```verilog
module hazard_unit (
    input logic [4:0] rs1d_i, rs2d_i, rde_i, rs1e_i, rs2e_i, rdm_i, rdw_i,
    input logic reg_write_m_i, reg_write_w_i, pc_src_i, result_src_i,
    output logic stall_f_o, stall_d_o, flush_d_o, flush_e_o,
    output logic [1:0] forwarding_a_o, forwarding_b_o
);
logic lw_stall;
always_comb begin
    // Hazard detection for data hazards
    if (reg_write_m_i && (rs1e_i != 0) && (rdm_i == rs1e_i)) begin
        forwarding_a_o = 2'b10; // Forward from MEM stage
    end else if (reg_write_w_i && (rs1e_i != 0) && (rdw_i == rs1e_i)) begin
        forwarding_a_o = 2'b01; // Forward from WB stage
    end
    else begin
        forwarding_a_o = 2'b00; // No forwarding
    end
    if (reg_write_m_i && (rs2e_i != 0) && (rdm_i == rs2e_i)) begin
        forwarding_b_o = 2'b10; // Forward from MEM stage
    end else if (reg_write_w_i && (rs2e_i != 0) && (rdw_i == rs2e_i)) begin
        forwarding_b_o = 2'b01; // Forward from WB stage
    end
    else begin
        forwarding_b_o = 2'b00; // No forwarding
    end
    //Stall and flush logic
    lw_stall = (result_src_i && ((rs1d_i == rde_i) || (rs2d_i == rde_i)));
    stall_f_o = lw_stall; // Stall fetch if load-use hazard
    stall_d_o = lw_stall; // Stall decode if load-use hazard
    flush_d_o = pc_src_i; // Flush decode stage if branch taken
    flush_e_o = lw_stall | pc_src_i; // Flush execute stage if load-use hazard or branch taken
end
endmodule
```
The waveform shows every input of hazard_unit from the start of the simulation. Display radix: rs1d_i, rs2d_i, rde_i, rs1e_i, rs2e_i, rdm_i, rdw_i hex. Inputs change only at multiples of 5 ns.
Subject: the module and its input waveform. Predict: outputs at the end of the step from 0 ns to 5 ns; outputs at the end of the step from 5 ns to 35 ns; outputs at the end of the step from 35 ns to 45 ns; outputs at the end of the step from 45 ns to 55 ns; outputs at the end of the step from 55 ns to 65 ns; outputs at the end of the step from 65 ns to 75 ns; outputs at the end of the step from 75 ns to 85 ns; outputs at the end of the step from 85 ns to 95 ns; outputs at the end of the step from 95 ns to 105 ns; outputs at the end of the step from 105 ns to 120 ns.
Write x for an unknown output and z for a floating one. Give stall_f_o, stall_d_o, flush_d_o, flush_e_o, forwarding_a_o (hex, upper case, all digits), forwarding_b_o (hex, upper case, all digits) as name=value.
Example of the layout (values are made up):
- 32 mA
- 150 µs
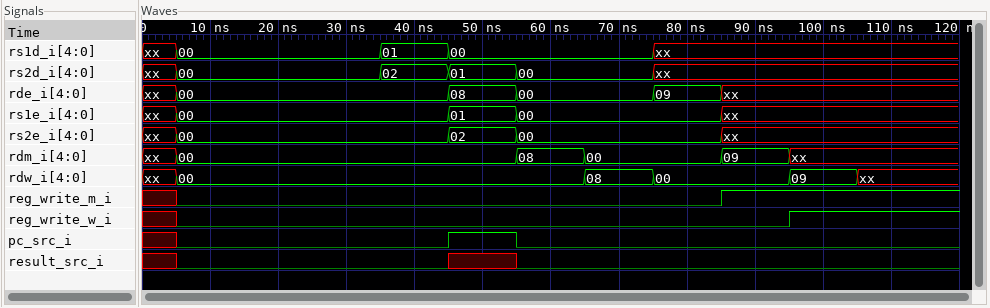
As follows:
- stall_f_o=x, stall_d_o=x, flush_d_o=x, flush_e_o=x, forwarding_a_o=0, forwarding_b_o=0
- stall_f_o=0, stall_d_o=0, flush_d_o=0, flush_e_o=0, forwarding_a_o=0, forwarding_b_o=0
- stall_f_o=0, stall_d_o=0, flush_d_o=0, flush_e_o=0, forwarding_a_o=0, forwarding_b_o=0
- stall_f_o=0, stall_d_o=0, flush_d_o=1, flush_e_o=1, forwarding_a_o=0, forwarding_b_o=0
- stall_f_o=0, stall_d_o=0, flush_d_o=0, flush_e_o=0, forwarding_a_o=0, forwarding_b_o=0
- stall_f_o=0, stall_d_o=0, flush_d_o=0, flush_e_o=0, forwarding_a_o=0, forwarding_b_o=0
- stall_f_o=0, stall_d_o=0, flush_d_o=0, flush_e_o=0, forwarding_a_o=0, forwarding_b_o=0
- stall_f_o=0, stall_d_o=0, flush_d_o=0, flush_e_o=0, forwarding_a_o=0, forwarding_b_o=0
- stall_f_o=0, stall_d_o=0, flush_d_o=0, flush_e_o=0, forwarding_a_o=0, forwarding_b_o=0
- stall_f_o=0, stall_d_o=0, flush_d_o=0, flush_e_o=0, forwarding_a_o=0, forwarding_b_o=0
